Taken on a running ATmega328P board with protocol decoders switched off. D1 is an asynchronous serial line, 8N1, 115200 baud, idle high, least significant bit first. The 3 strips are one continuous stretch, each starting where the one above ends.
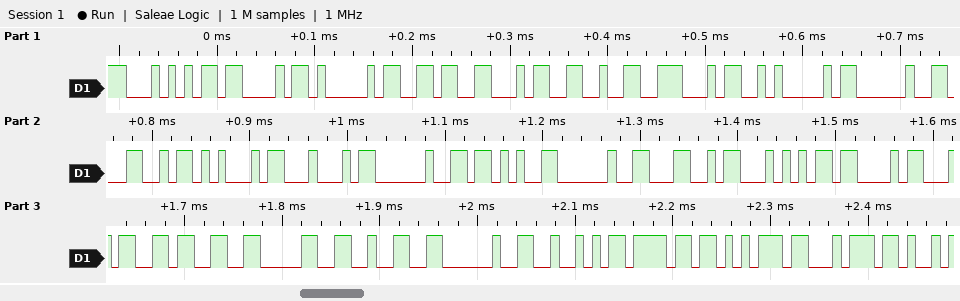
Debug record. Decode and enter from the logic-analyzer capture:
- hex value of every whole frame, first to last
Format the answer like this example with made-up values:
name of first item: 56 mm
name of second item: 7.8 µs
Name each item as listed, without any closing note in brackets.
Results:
hex value of every whole frame, first to last: 54 43 41 36 34 32 34 41 20 4C 45 44 20 2B 20 4C 54 43 34 33 30 32 20 52 6F 75 74
